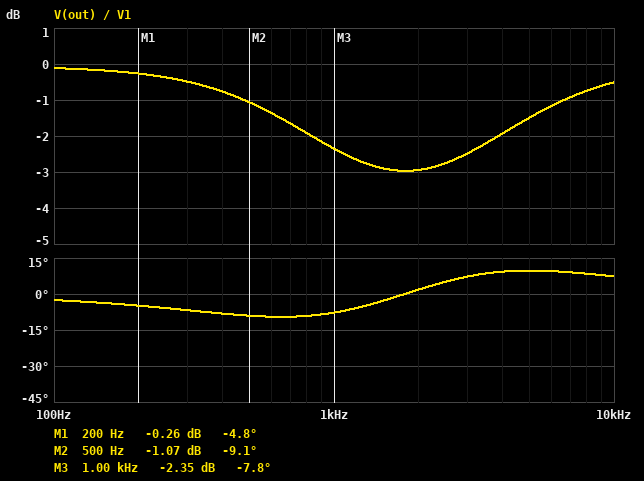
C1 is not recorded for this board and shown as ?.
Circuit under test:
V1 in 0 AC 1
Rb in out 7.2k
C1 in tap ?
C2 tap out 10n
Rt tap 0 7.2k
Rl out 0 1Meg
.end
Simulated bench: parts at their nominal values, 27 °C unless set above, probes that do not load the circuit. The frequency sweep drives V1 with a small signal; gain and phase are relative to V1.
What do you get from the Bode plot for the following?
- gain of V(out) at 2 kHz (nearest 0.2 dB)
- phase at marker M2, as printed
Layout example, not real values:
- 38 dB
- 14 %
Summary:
- -3.0 dB
- -9.1 deg
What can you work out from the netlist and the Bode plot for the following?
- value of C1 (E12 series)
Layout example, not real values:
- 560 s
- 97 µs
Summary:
- 15 nF
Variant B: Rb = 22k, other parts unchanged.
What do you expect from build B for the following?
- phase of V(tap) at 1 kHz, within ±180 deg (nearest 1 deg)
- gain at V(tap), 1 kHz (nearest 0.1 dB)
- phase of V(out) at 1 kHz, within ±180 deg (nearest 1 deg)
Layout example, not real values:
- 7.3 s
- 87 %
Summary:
- 41 deg
- -4.7 dB
- -1 deg
